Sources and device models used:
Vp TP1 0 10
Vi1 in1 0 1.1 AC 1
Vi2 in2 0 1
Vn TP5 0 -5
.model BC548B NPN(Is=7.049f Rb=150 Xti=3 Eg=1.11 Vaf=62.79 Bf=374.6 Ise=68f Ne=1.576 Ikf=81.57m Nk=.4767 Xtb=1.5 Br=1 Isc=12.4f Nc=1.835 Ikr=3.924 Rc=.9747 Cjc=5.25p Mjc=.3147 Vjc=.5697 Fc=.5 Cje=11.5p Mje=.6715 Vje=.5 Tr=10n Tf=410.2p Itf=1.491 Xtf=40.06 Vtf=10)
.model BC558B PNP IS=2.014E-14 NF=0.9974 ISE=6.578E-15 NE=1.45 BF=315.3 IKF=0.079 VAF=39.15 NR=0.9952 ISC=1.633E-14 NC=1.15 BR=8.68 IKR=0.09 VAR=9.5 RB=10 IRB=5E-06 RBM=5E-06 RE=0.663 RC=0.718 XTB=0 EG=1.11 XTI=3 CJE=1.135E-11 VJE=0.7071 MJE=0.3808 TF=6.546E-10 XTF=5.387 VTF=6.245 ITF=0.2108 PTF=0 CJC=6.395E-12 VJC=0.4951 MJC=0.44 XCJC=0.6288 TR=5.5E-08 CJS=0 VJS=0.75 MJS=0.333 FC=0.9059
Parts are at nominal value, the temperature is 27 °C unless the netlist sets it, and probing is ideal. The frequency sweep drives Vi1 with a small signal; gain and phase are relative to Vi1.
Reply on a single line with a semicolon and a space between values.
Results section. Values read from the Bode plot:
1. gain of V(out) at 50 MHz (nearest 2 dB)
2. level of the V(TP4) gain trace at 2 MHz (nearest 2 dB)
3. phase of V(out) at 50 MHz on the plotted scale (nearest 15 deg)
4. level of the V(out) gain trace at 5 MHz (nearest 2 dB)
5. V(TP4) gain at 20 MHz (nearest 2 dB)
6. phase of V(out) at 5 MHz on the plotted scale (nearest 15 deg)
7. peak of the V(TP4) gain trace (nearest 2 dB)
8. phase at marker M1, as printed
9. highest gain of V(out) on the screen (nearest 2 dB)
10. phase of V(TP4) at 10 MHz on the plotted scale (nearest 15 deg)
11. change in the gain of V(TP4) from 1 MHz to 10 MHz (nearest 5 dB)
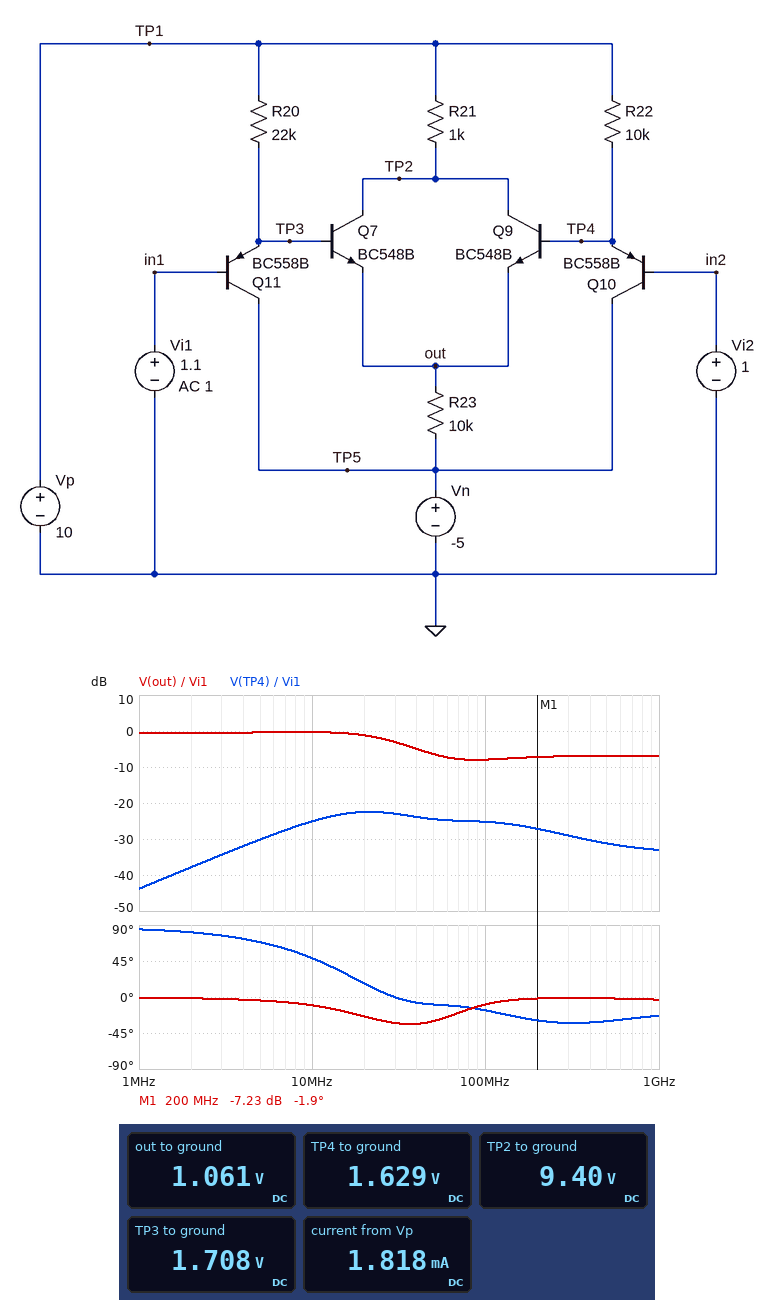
-6 dB; -38 dB; -30 deg; 0 dB; -22 dB; 0 deg; -22 dB; -1.9 deg; 0 dB; 45 deg; 20 dB
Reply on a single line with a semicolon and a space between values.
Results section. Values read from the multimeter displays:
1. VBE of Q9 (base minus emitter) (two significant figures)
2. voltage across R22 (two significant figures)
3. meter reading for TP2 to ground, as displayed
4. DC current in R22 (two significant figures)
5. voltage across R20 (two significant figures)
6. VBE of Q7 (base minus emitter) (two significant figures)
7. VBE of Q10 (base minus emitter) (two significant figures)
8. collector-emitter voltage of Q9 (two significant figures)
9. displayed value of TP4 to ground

570 mV; 8.4 V; 9.40 V; 840 µA; 8.3 V; 650 mV; -630 mV; 8.3 V; 1.629 V
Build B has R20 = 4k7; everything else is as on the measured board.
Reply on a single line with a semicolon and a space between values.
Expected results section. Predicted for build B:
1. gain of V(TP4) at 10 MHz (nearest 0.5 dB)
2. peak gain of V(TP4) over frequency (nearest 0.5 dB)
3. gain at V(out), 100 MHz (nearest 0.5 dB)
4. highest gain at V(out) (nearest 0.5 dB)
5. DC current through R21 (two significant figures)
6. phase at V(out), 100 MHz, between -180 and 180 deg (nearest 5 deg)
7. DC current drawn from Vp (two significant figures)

-25.5 dB; -22.0 dB; -7.5 dB; 0 dB; 610 µA; -15 deg; 3.2 mA
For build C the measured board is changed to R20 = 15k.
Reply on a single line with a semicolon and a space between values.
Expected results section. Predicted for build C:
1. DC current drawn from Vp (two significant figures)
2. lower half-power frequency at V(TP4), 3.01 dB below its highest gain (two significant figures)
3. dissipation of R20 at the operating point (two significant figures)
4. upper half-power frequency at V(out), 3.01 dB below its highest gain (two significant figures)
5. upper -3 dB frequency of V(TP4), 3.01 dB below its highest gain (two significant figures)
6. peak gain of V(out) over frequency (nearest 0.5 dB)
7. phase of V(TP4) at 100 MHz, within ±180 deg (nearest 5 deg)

2.0 mA; 9.8 MHz; 4.6 mW; 33 MHz; 110 MHz; 0 dB; -20 deg
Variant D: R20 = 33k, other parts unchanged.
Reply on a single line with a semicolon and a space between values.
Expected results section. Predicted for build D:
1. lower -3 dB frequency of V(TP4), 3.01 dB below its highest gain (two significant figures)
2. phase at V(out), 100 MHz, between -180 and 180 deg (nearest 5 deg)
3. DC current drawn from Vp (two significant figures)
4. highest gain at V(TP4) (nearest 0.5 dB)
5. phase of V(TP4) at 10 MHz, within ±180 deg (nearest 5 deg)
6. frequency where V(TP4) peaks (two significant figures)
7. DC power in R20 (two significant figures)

8.9 MHz; -5 deg; 1.7 mA; -23.0 dB; 45 deg; 20 MHz; 2.1 mW
